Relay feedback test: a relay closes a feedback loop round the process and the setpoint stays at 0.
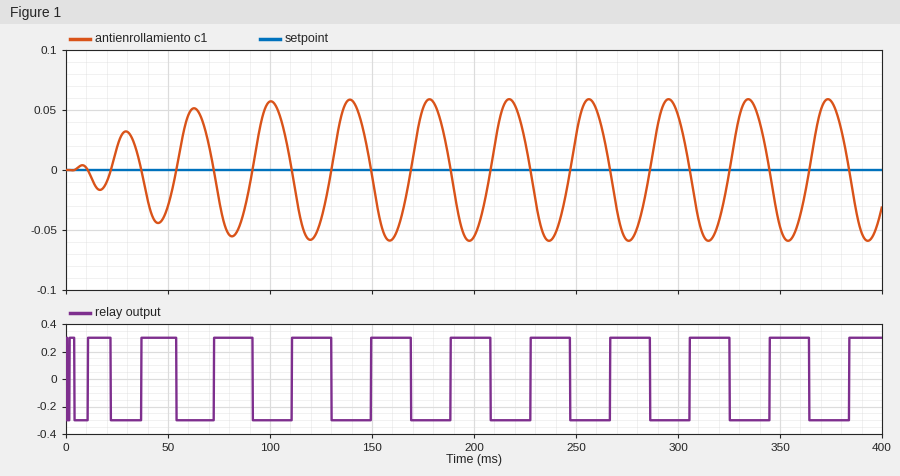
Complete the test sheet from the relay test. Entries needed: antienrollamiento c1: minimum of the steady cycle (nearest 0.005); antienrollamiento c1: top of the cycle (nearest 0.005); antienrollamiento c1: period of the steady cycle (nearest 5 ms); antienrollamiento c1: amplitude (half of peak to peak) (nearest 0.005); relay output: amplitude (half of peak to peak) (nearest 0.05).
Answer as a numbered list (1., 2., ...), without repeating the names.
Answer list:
1. -0.060
2. 0.060
3. 40 ms
4. 0.060
5. 0.30
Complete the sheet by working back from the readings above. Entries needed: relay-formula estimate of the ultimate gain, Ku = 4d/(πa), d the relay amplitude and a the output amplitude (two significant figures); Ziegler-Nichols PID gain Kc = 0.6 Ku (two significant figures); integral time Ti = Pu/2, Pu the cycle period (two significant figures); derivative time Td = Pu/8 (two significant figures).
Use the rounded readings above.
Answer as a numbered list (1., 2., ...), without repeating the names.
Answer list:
1. 6.4
2. 3.8
3. 20 ms
4. 5.0 ms
